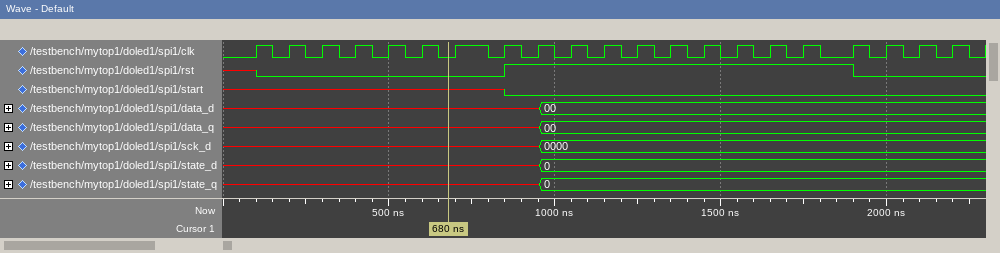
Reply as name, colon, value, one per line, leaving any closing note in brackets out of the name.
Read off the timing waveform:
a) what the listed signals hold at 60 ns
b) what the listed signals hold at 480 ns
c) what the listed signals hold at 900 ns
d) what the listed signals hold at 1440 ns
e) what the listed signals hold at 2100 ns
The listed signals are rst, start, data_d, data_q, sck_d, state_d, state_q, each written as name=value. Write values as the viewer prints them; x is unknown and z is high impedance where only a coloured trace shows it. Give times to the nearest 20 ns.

what the listed signals hold at 60 ns: rst=x, start=x, data_d=x, data_q=x, sck_d=x, state_d=x, state_q=x
what the listed signals hold at 480 ns: rst=0, start=x, data_d=x, data_q=x, sck_d=x, state_d=x, state_q=x
what the listed signals hold at 900 ns: rst=1, start=0, data_d=x, data_q=x, sck_d=x, state_d=x, state_q=x
what the listed signals hold at 1440 ns: rst=1, start=0, data_d=00, data_q=00, sck_d=0000, state_d=0, state_q=0
what the listed signals hold at 2100 ns: rst=0, start=0, data_d=00, data_q=00, sck_d=0000, state_d=0, state_q=0
